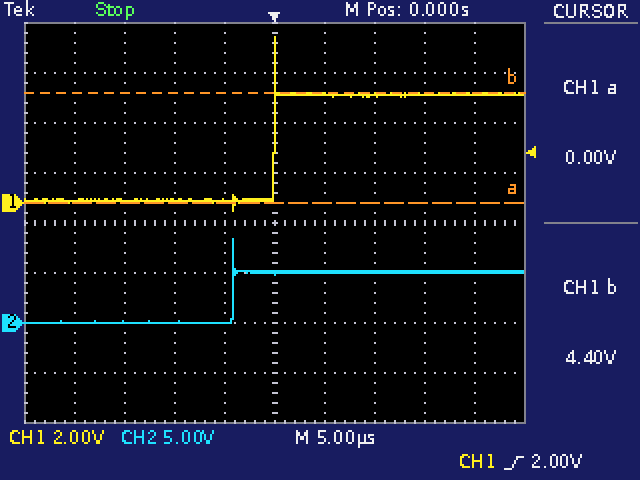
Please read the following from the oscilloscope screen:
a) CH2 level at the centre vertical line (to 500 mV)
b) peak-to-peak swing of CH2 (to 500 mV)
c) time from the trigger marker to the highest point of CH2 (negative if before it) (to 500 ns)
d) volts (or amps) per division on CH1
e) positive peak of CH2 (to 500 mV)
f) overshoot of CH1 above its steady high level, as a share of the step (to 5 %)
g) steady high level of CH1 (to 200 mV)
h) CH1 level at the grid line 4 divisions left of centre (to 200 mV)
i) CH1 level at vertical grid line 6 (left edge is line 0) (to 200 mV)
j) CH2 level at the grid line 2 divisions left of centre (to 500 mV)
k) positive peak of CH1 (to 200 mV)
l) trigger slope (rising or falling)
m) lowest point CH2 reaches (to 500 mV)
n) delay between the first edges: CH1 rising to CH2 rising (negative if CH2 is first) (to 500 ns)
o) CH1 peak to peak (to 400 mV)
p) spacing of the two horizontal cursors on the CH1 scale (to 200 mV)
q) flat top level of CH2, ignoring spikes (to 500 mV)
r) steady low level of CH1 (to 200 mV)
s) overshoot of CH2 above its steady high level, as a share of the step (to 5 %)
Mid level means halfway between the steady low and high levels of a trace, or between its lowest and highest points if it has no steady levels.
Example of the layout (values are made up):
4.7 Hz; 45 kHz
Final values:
5.0 V; 8.5 V; -4.0 µs; 2 V; 8.5 V; 55 %; 4.4 V; 0.0 V; 4.4 V; 0.0 V; 6.6 V; rising; 0.0 V; -4.0 µs; 6.8 V; 4.4 V; 5.0 V; 0.0 V; 65 %
